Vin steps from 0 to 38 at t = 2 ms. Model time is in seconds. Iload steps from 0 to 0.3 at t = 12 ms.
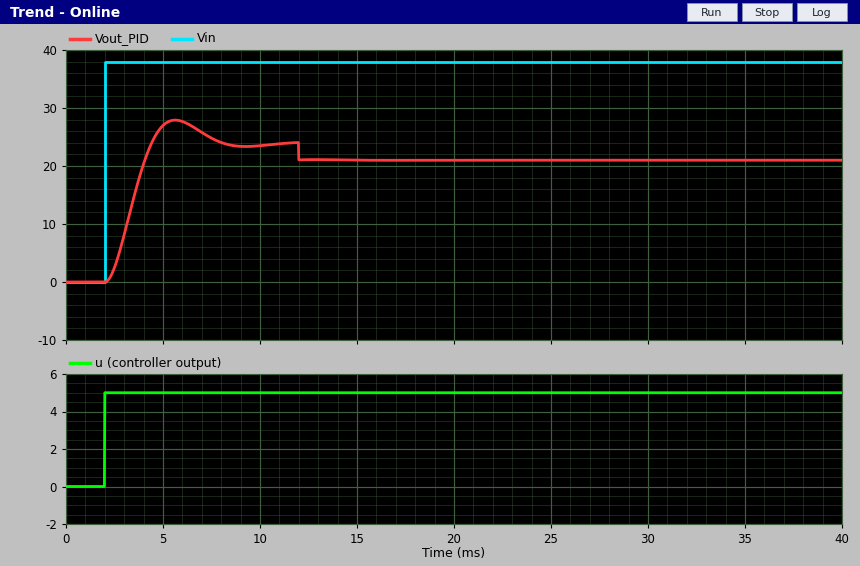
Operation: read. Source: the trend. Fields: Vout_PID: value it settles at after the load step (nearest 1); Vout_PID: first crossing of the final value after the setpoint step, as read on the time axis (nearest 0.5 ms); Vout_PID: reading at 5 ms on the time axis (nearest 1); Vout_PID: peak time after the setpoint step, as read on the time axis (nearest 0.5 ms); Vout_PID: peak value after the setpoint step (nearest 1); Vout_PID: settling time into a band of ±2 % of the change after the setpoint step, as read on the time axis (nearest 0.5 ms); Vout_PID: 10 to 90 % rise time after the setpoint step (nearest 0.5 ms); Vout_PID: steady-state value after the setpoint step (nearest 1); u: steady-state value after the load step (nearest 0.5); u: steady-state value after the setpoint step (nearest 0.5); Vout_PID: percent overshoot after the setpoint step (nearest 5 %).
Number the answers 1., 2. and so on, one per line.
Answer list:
1. 21
2. 4.5 ms
3. 27
4. 5.5 ms
5. 28
6. 10.0 ms
7. 1.5 ms
8. 24
9. 5.0
10. 5.0
11. 15 %
